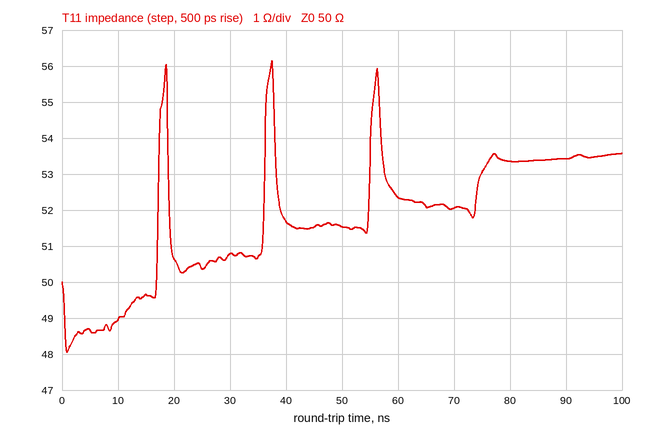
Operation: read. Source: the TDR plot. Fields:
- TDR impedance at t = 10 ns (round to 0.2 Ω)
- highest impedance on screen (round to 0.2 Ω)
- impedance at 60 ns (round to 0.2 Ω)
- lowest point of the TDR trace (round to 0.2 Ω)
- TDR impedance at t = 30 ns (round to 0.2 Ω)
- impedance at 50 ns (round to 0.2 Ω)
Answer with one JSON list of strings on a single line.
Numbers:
["49.0 Ω", "56.2 Ω", "52.4 Ω", "48.0 Ω", "50.8 Ω", "51.6 Ω"]
